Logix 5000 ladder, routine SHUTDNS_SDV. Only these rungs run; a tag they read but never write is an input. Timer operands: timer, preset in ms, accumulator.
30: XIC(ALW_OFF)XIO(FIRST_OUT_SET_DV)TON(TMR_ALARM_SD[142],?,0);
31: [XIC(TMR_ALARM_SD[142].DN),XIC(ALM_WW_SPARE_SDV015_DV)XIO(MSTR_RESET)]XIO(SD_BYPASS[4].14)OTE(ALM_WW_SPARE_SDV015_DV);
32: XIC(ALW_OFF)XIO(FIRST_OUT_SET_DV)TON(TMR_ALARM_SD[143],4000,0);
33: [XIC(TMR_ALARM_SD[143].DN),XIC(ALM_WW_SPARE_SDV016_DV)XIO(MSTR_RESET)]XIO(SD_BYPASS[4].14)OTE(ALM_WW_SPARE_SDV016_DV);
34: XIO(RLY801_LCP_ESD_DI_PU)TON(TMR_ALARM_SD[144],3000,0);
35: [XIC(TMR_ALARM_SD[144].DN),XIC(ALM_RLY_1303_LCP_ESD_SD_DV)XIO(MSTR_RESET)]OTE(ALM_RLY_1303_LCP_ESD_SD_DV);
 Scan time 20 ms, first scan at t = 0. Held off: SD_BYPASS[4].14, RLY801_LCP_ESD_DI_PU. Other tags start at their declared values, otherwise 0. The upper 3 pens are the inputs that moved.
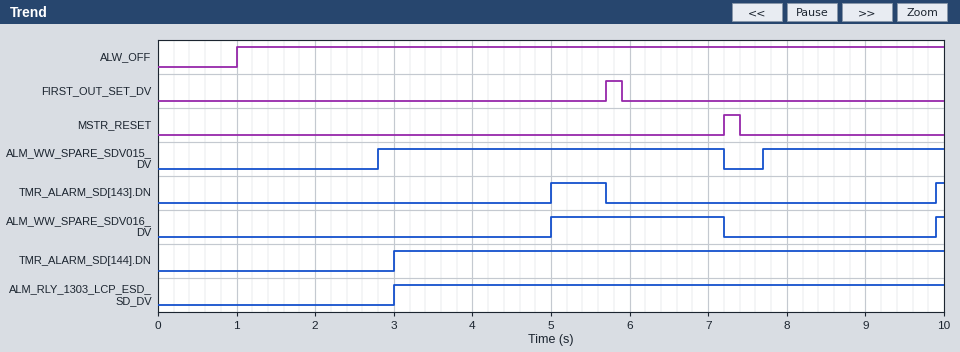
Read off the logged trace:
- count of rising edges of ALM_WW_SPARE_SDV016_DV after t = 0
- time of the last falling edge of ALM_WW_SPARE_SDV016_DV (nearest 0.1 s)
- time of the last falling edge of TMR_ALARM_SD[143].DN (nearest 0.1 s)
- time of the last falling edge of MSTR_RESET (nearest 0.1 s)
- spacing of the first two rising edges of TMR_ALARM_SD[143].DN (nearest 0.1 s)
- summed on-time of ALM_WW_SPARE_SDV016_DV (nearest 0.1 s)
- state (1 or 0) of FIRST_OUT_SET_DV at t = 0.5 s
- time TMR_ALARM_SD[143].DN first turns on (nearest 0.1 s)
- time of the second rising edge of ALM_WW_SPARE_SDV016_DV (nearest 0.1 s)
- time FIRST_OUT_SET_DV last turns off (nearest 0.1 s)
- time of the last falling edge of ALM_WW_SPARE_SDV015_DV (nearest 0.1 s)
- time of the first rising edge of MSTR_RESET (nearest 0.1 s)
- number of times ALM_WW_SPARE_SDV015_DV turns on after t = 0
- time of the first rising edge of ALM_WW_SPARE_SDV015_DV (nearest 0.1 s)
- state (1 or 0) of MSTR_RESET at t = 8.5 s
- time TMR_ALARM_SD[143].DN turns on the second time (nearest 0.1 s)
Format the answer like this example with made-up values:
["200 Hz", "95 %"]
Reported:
["2", "7.2 s", "5.7 s", "7.4 s", "4.9 s", "2.3 s", "0", "5.0 s", "9.9 s", "5.9 s", "7.2 s", "7.2 s", "2", "2.8 s", "0", "9.9 s"]
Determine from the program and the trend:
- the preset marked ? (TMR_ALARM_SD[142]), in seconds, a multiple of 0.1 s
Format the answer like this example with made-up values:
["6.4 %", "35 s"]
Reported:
["1.8 s"]
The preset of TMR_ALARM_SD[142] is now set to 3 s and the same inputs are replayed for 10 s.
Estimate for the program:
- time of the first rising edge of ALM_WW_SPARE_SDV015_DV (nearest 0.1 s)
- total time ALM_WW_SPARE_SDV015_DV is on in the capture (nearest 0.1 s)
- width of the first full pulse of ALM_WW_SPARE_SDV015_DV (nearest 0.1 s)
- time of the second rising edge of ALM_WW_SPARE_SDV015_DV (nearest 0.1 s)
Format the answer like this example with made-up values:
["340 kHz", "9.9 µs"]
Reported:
["4.0 s", "4.3 s", "3.2 s", "8.9 s"]
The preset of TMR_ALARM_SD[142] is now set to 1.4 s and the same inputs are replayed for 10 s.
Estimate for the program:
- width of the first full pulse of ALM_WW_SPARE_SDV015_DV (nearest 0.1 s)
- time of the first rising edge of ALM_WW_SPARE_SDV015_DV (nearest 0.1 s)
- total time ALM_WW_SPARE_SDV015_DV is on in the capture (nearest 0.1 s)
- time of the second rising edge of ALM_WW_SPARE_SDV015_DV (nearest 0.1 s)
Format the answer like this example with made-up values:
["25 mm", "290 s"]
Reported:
["4.8 s", "2.4 s", "7.5 s", "7.3 s"]
